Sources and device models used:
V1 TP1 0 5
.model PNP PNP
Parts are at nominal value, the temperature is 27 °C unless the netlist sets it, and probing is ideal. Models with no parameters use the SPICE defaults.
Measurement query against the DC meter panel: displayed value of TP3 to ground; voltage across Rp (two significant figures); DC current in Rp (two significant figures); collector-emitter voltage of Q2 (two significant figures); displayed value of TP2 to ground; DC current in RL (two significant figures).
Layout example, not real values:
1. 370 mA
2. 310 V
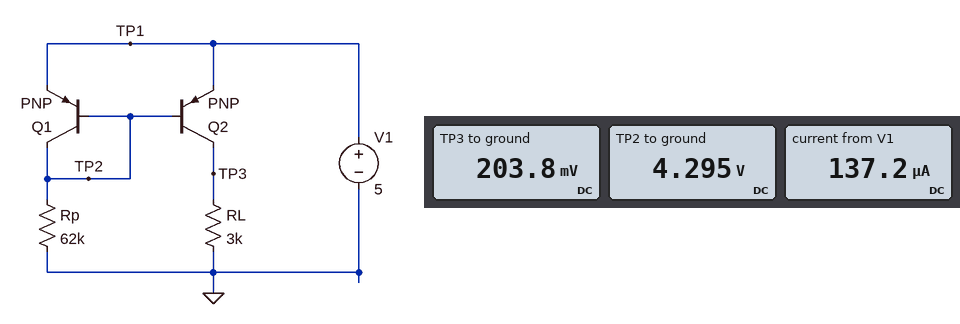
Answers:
1. 203.8 mV
2. 4.3 V
3. 69 µA
4. -4.8 V
5. 4.295 V
6. 68 µA
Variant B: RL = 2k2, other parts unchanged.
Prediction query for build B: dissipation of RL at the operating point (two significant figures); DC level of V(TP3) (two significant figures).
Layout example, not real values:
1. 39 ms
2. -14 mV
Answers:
1. 10 µW
2. 150 mV
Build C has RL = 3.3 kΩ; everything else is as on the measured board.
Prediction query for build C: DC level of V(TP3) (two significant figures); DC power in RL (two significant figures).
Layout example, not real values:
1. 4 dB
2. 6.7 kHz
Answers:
1. 220 mV
2. 15 µW
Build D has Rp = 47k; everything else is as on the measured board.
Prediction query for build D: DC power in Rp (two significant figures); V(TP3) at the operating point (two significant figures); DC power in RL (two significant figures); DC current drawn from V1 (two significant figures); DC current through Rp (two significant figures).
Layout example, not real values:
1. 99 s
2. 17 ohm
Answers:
1. 390 µW
2. 270 mV
3. 24 µW
4. 180 µA
5. 91 µA
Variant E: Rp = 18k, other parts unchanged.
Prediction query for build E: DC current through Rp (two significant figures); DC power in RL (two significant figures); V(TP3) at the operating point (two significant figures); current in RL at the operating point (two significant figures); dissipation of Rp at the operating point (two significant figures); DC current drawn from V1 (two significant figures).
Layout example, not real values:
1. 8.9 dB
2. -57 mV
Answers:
1. 240 µA
2. 160 µW
3. 700 mV
4. 230 µA
5. 1.0 mW
6. 470 µA
